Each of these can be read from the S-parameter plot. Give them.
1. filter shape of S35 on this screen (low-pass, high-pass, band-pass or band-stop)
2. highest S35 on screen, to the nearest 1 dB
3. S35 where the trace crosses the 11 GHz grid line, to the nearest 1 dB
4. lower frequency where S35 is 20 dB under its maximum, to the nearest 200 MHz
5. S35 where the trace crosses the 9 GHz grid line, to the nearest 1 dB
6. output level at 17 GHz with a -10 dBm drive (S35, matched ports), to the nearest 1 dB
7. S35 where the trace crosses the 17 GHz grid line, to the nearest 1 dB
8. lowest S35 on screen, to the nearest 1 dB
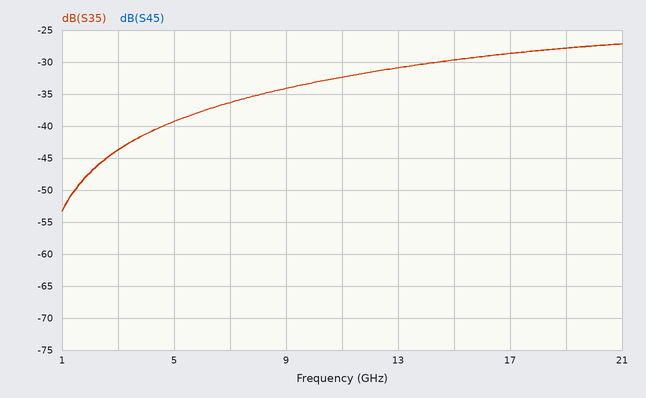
high-pass
-27 dB
-32 dB
2.0 GHz
-34 dB
-39 dBm
-29 dB
-53 dB
